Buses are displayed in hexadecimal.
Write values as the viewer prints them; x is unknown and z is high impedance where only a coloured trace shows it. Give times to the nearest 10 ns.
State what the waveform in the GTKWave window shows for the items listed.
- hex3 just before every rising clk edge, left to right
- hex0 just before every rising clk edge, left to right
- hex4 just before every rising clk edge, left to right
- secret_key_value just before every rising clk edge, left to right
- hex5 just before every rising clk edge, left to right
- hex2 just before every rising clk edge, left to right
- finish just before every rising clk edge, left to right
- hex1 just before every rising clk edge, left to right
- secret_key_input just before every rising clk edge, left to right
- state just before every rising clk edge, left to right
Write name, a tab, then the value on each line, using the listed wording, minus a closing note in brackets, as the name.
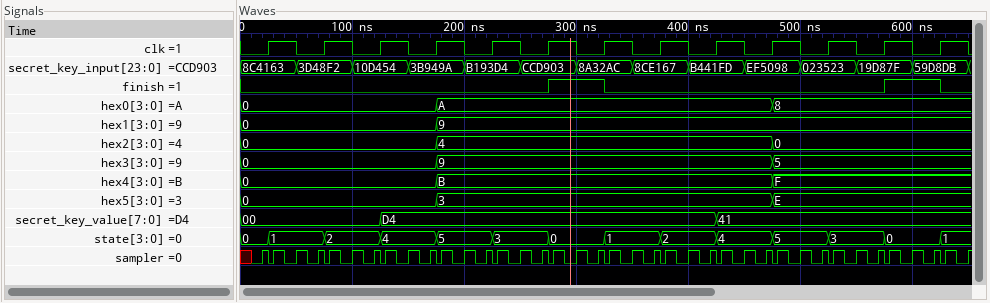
hex3 just before every rising clk edge, left to right	0, 0, 0, 0, 9, 9, 9, 9, 9, 9, 5, 5, 5
hex0 just before every rising clk edge, left to right	0, 0, 0, 0, A, A, A, A, A, A, 8, 8, 8
hex4 just before every rising clk edge, left to right	0, 0, 0, 0, B, B, B, B, B, B, F, F, F
secret_key_value just before every rising clk edge, left to right	00, 00, 00, D4, D4, D4, D4, D4, D4, 41, 41, 41, 41
hex5 just before every rising clk edge, left to right	0, 0, 0, 0, 3, 3, 3, 3, 3, 3, E, E, E
hex2 just before every rising clk edge, left to right	0, 0, 0, 0, 4, 4, 4, 4, 4, 4, 0, 0, 0
finish just before every rising clk edge, left to right	0 0 0 0 0 0 1 0 0 0 0 0 1
hex1 just before every rising clk edge, left to right	0, 0, 0, 0, 9, 9, 9, 9, 9, 9, 9, 9, 9
secret_key_input just before every rising clk edge, left to right	8C4163, 3D48F2, 10D454, 3B949A, B193D4, CCD903, 8A32AC, 8CE167, B441FD, EF5098, 023523, 19D87F, 59D8DB
state just before every rising clk edge, left to right	0, 1, 2, 4, 5, 3, 0, 1, 2, 4, 5, 3, 0
